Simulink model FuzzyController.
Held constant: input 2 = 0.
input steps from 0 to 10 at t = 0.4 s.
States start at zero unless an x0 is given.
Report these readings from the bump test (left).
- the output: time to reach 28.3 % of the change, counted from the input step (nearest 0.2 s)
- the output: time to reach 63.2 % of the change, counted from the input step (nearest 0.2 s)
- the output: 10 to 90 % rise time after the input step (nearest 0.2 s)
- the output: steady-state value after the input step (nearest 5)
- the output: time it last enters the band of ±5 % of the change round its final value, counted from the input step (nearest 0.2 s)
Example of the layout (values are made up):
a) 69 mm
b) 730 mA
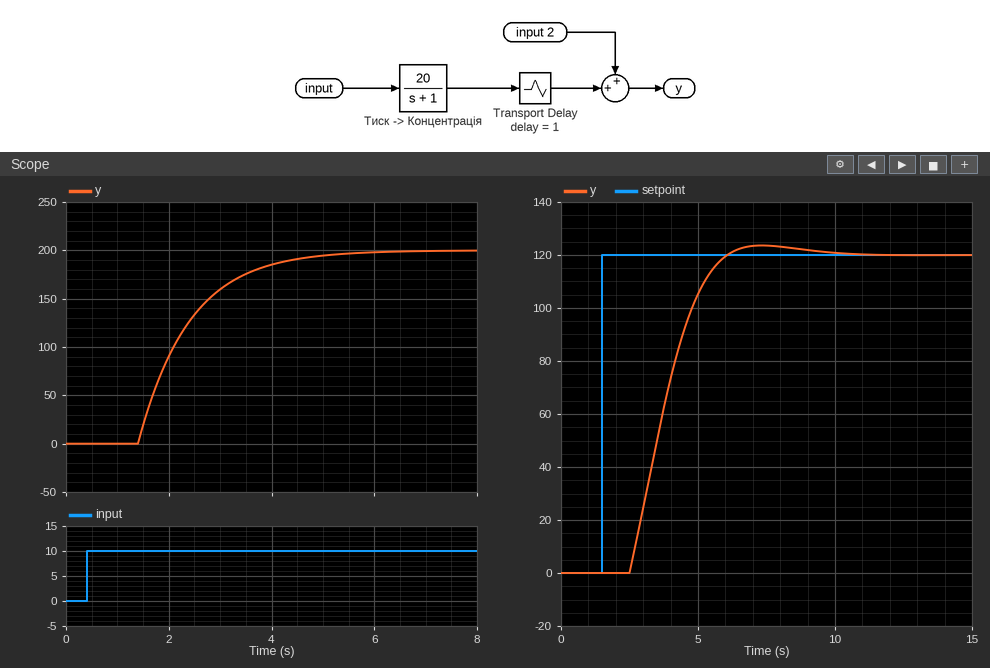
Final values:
a) 1.4 s
b) 2.0 s
c) 2.2 s
d) 200
e) 4.0 s
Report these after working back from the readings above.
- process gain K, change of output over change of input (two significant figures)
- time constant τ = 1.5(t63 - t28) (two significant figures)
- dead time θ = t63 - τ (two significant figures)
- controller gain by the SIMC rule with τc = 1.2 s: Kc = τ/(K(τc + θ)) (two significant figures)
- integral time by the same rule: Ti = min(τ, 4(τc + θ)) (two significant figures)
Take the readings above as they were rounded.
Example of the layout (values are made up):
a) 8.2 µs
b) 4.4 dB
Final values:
a) 20
b) 0.90 s
c) 1.1 s
d) 0.020
e) 0.90 s
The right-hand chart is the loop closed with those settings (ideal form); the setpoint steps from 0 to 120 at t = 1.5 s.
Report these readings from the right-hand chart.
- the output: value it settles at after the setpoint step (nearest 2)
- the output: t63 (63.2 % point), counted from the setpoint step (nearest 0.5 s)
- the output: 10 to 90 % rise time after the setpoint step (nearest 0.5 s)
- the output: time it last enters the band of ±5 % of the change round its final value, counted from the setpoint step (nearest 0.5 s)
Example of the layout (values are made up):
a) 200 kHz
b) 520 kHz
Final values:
a) 120
b) 2.5 s
c) 2.5 s
d) 4.0 s
